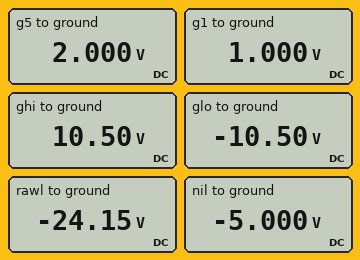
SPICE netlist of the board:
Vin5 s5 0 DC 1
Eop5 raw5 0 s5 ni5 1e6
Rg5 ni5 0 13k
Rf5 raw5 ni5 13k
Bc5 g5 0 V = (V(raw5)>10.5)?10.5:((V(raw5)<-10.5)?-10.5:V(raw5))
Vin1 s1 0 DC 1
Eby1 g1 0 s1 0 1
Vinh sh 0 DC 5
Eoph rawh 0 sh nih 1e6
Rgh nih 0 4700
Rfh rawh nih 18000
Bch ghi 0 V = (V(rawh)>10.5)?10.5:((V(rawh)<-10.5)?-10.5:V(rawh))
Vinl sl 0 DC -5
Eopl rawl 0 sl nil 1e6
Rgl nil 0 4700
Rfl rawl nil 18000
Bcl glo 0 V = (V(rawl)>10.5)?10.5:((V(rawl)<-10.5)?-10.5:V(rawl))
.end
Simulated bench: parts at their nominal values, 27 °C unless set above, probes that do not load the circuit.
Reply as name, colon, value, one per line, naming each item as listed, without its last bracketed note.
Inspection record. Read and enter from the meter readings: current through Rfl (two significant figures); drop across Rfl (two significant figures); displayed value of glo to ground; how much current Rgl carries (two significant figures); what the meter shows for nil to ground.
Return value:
current through Rfl: 1.1 mA
drop across Rfl: 19 V
displayed value of glo to ground: -10.50 V
how much current Rgl carries: 1.1 mA
what the meter shows for nil to ground: -5.000 V
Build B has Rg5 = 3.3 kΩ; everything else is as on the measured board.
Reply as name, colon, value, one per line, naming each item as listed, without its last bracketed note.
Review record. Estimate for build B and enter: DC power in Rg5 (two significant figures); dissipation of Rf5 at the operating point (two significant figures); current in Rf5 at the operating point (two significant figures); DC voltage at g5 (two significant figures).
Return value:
DC power in Rg5: 300 µW
dissipation of Rf5 at the operating point: 1.2 mW
current in Rf5 at the operating point: 300 µA
DC voltage at g5: 4.9 V
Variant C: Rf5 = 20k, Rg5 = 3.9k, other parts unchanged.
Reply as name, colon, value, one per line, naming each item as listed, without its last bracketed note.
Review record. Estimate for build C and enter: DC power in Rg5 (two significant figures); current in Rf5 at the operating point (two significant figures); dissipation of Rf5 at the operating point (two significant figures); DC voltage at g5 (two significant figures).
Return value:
DC power in Rg5: 260 µW
current in Rf5 at the operating point: 260 µA
dissipation of Rf5 at the operating point: 1.3 mW
DC voltage at g5: 6.1 V
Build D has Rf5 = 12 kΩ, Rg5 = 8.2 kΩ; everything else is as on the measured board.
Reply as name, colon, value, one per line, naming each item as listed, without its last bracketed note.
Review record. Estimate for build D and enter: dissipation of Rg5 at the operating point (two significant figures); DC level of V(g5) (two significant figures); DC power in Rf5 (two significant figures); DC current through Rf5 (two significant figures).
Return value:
dissipation of Rg5 at the operating point: 120 µW
DC level of V(g5): 2.5 V
DC power in Rf5: 180 µW
DC current through Rf5: 120 µA
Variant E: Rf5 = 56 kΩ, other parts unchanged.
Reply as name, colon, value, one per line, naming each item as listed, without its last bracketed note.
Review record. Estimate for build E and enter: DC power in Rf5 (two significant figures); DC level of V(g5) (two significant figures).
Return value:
DC power in Rf5: 330 µW
DC level of V(g5): 5.3 V
